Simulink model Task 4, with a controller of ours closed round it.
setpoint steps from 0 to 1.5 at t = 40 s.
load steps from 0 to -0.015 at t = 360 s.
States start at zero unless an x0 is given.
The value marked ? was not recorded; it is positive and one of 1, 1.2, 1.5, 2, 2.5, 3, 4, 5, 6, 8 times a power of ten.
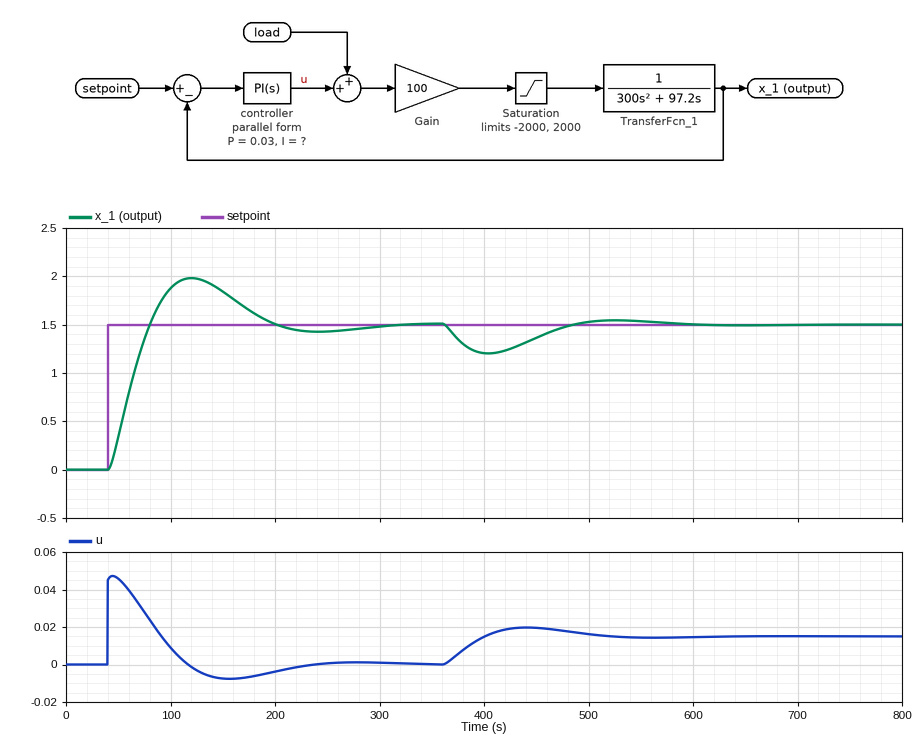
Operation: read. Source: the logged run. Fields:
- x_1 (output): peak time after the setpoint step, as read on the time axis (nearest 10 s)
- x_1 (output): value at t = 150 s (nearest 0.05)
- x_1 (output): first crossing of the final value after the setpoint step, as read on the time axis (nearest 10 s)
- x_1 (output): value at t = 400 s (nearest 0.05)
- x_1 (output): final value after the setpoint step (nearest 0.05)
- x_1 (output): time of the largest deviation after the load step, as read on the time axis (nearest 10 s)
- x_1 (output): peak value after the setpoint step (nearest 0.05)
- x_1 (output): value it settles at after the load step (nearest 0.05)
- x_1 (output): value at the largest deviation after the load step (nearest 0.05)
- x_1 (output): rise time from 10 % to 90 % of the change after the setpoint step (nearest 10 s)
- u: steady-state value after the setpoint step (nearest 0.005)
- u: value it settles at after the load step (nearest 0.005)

120 s
1.85
80 s
1.20
1.50
400 s
2.00
1.50
1.20
30 s
0.000
0.015
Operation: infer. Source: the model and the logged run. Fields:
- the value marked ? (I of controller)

0.0008
